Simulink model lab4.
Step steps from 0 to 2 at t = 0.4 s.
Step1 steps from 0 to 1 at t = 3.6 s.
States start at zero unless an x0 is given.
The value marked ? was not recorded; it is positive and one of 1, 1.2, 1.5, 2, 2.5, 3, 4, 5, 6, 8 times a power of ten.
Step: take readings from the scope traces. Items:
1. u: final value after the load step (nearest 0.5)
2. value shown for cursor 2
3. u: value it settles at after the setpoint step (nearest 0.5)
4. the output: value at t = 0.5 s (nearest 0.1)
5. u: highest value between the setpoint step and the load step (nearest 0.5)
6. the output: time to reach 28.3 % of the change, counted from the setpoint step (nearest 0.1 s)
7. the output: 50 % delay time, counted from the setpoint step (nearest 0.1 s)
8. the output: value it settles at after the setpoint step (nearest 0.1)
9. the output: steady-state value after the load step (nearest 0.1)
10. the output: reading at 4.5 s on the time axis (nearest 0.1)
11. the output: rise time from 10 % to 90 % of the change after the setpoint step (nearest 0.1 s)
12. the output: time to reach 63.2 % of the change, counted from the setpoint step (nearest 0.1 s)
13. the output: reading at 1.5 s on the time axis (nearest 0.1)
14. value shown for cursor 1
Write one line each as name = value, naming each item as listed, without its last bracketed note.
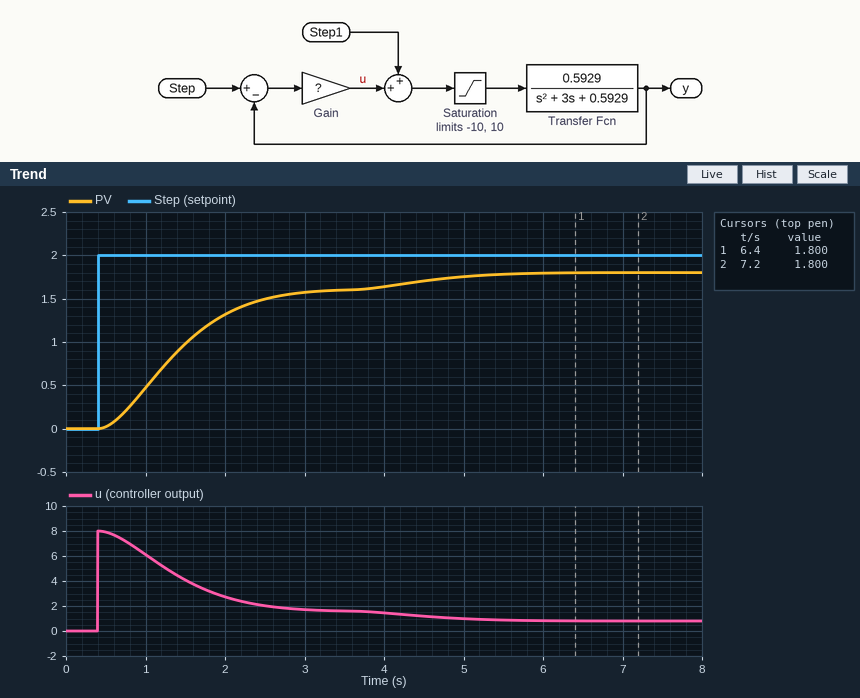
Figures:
u: final value after the load step = 1.0
value shown for cursor 2 = 1.800
u: value it settles at after the setpoint step = 1.5
the output: value at t = 0.5 s = 0.0
u: highest value between the setpoint step and the load step = 8.0
the output: time to reach 28.3 % of the change, counted from the setpoint step = 0.6 s
the output: 50 % delay time, counted from the setpoint step = 0.9 s
the output: value it settles at after the setpoint step = 1.6
the output: steady-state value after the load step = 1.8
the output: reading at 4.5 s on the time axis = 1.7
the output: rise time from 10 % to 90 % of the change after the setpoint step = 1.6 s
the output: time to reach 63.2 % of the change, counted from the setpoint step = 1.1 s
the output: reading at 1.5 s on the time axis = 1.0
value shown for cursor 1 = 1.800
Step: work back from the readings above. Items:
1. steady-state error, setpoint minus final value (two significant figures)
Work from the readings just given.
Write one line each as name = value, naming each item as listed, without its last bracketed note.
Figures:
steady-state error, setpoint minus final value = 0.40
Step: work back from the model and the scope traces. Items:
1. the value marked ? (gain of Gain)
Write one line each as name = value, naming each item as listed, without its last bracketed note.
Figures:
the value marked ? = 4
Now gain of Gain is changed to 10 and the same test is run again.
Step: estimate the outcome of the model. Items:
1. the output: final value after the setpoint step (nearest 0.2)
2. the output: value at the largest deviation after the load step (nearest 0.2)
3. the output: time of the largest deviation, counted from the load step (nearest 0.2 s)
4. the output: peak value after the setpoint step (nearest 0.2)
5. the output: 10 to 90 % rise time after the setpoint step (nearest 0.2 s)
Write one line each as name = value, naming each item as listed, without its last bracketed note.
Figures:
the output: final value after the setpoint step = 1.8
the output: value at the largest deviation after the load step = 2.0
the output: time of the largest deviation, counted from the load step = 1.6 s
the output: peak value after the setpoint step = 2.0
the output: 10 to 90 % rise time after the setpoint step = 1.0 s
